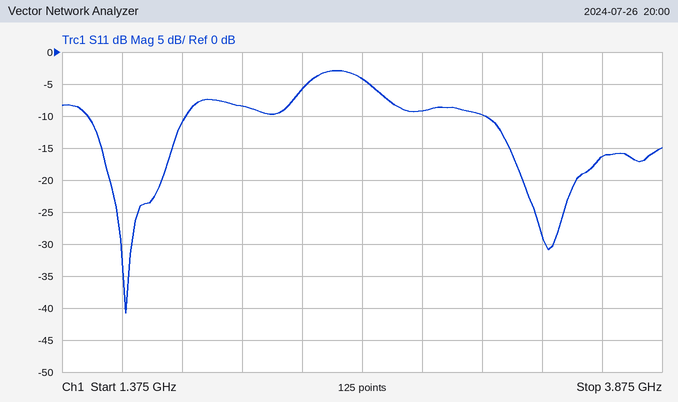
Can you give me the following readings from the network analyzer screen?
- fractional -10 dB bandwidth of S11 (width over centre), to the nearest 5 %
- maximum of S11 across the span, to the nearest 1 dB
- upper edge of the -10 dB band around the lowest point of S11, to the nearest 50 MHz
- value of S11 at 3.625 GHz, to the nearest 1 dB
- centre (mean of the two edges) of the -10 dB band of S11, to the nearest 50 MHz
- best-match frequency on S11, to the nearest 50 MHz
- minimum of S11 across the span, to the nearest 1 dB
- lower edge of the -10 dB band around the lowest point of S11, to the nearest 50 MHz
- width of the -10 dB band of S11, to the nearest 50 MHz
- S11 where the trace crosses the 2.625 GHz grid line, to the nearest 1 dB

25 %
-3 dB
1.90 GHz
-16 dB
1.70 GHz
1.65 GHz
-41 dB
1.50 GHz
400 MHz
-4 dB
